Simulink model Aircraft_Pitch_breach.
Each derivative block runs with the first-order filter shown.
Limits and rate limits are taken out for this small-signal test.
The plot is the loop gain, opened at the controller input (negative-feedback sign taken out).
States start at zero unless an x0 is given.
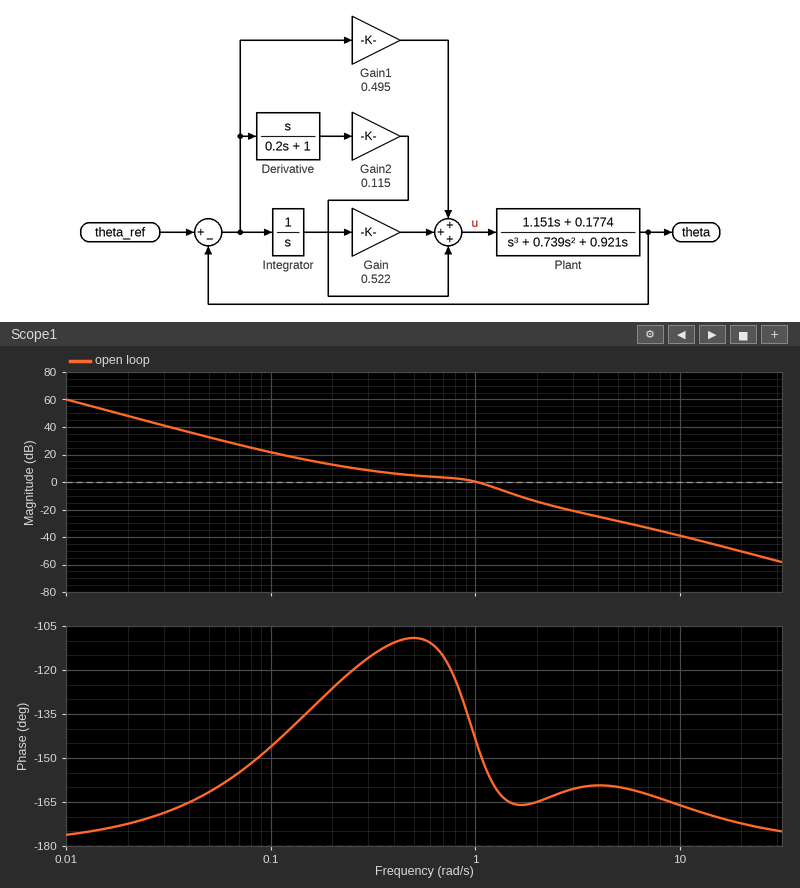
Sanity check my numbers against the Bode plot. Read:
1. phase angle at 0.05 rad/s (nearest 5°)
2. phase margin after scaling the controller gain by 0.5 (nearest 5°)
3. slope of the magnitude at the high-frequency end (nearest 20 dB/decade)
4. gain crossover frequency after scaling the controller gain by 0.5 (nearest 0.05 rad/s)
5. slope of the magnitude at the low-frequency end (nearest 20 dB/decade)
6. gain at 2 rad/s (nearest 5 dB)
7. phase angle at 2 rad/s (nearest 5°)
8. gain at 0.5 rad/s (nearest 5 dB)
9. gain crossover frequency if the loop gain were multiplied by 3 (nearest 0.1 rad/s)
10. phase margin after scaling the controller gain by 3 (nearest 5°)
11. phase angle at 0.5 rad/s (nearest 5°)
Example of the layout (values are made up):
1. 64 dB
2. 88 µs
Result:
1. -160°
2. 70°
3. -40 dB/decade
4. 0.40 rad/s
5. -40 dB/decade
6. -15 dB
7. -165°
8. 5 dB
9. 1.6 rad/s
10. 15°
11. -110°
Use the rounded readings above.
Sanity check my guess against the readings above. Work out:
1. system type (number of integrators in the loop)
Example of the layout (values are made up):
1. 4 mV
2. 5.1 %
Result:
1. 2
